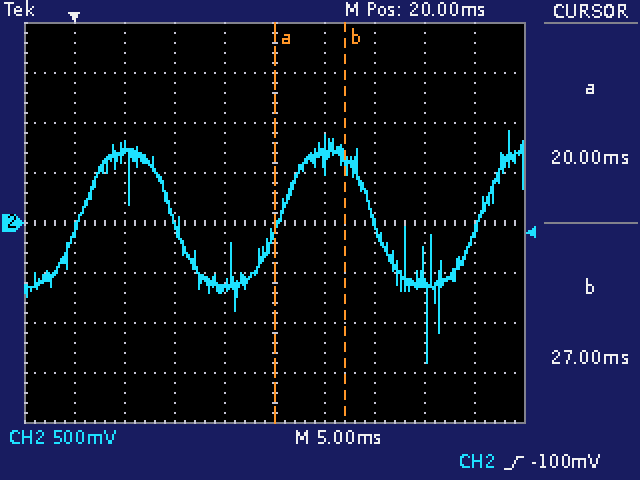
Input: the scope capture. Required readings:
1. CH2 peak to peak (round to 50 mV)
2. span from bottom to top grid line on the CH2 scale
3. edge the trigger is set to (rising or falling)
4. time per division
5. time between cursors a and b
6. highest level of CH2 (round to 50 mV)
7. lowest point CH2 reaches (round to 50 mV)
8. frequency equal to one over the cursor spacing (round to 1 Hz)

2.30 V
4 V
rising
5 ms
7.0 ms
900 mV
-1.40 V
143 Hz
